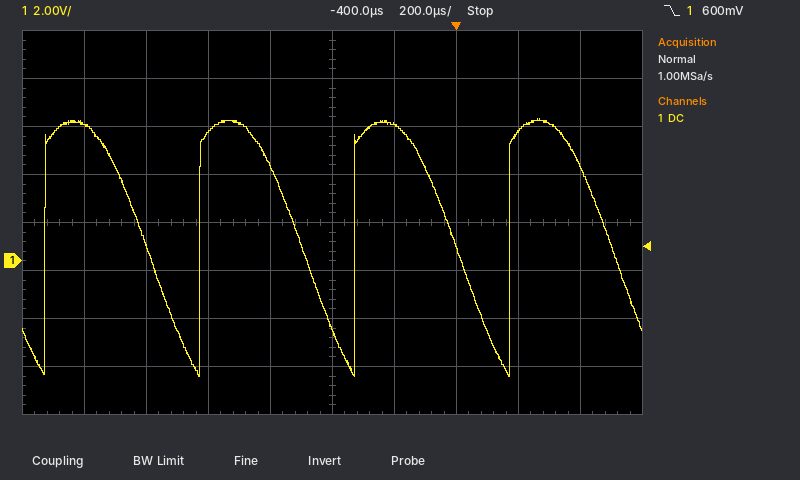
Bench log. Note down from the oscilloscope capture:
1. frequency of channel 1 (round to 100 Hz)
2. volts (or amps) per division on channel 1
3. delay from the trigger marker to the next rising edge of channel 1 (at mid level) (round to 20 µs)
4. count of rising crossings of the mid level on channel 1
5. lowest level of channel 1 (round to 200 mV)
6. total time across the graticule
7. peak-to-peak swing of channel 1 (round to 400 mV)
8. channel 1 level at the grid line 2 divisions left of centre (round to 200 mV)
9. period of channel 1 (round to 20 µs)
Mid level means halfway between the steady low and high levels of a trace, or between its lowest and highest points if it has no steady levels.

2.0 kHz
2 V
180 µs
4
-4.8 V
2 ms
10.8 V
5.4 V
500 µs
